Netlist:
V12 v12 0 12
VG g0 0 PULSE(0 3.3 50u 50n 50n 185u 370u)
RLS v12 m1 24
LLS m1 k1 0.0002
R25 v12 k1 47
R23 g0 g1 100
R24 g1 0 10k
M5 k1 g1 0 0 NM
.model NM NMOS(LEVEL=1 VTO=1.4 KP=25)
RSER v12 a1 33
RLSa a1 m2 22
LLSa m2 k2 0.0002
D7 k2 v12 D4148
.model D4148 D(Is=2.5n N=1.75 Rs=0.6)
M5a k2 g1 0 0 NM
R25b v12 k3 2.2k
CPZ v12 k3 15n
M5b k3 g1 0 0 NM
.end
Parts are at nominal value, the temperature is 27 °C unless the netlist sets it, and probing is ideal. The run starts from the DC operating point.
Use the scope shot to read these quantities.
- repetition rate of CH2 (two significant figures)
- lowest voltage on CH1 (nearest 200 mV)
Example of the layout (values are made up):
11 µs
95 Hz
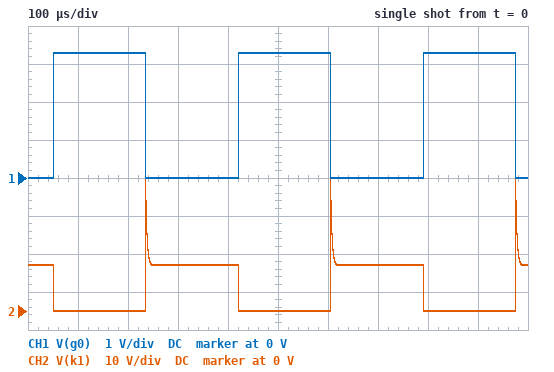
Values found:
2.7 kHz
0 V
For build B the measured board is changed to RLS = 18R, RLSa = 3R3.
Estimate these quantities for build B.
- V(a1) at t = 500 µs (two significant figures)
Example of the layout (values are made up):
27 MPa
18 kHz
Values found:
1.1 V
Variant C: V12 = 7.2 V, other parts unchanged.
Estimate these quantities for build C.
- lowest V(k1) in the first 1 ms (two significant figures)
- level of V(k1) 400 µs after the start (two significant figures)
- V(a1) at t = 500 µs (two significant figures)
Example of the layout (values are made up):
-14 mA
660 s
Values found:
3.3 mV
7.2 V
2.9 V
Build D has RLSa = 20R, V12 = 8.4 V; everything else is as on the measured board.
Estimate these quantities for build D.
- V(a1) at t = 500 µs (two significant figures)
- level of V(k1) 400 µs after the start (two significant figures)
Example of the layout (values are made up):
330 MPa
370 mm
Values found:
3.2 V
8.4 V
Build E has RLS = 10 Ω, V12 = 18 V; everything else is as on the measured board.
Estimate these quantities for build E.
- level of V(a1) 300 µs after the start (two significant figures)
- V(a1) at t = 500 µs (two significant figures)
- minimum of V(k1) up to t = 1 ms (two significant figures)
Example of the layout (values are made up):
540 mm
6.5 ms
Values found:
18 V
7.2 V
8.3 mV
